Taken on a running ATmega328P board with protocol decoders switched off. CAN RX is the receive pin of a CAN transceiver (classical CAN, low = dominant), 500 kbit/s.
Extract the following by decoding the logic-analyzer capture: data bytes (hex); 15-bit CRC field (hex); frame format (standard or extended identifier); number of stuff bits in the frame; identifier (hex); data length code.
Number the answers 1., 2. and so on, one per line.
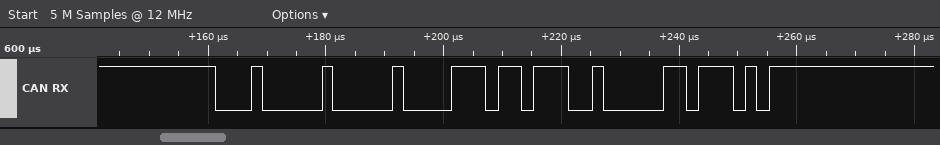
1. DB
2. 0x482E
3. standard
4. 3
5. 0x100
6. 1
